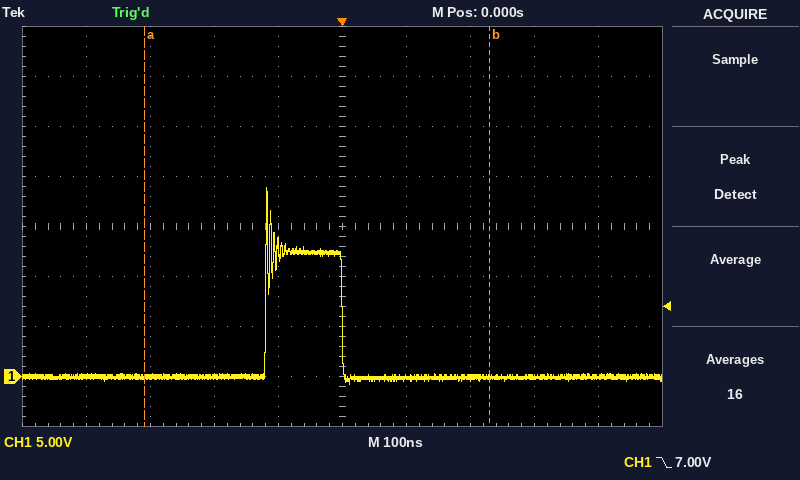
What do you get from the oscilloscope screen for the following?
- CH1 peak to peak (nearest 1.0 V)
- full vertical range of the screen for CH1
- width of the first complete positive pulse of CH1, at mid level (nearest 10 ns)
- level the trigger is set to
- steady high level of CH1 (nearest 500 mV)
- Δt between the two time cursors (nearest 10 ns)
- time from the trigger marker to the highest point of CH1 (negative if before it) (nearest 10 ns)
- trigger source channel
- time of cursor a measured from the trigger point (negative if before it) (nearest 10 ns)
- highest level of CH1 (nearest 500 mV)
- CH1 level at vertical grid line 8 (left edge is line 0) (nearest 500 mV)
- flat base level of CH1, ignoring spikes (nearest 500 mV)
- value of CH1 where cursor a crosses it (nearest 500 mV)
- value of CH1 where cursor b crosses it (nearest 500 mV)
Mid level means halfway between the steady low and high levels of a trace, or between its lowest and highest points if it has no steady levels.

20.0 V
40 V
120 ns
7.00 V
12.5 V
540 ns
-120 ns
CH1
-310 ns
19.0 V
0.0 V
0.0 V
0.0 V
0.0 V
